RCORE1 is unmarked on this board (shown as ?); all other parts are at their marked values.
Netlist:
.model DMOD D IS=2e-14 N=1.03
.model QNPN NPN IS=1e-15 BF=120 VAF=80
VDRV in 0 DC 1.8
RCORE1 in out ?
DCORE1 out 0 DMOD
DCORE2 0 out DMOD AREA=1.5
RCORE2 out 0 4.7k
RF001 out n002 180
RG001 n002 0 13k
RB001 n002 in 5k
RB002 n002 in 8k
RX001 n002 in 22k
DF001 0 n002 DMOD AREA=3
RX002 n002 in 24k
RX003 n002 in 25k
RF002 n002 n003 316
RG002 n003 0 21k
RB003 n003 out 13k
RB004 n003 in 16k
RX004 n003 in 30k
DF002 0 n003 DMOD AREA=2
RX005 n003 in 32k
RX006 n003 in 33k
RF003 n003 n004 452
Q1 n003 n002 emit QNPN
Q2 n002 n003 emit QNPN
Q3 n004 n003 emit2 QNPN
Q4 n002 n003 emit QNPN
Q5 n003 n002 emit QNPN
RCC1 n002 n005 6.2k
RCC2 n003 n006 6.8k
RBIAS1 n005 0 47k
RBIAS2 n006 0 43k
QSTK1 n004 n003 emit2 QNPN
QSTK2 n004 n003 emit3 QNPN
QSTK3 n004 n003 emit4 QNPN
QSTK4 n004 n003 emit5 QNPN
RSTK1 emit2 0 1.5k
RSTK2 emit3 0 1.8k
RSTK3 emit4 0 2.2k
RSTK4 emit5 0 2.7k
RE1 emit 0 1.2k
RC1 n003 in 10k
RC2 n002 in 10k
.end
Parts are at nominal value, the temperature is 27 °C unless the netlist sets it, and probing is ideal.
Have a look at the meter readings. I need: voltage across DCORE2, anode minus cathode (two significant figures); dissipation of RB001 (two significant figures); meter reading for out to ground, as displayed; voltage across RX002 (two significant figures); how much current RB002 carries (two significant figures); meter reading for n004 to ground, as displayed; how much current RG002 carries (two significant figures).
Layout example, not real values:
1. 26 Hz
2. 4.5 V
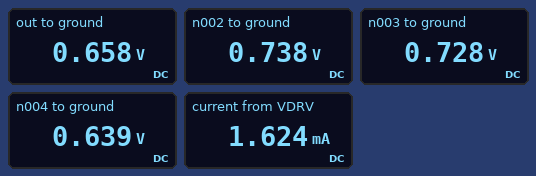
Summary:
1. -660 mV
2. 230 µW
3. 0.658 V
4. 1.1 V
5. 130 µA
6. 0.639 V
7. 35 µA
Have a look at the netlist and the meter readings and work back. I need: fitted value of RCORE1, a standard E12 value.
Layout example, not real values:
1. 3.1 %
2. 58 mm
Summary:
1. 1.5 kΩ
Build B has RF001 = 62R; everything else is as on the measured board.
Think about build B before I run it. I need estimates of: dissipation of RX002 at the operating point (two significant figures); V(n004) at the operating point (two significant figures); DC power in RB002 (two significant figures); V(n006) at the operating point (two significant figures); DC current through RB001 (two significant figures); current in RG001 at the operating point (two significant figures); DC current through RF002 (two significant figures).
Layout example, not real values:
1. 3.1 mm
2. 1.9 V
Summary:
1. 51 µW
2. 630 mV
3. 150 µW
4. 610 mV
5. 220 µA
6. 53 µA
7. 39 µA
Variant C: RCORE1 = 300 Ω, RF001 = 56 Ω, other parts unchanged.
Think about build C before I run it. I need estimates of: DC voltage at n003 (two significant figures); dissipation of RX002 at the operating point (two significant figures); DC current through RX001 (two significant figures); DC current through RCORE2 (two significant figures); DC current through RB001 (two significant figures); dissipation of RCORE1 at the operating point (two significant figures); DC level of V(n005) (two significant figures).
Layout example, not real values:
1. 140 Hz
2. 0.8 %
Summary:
1. 720 mV
2. 49 µW
3. 49 µA
4. 150 µA
5. 220 µA
6. 4.1 mW
7. 640 mV
